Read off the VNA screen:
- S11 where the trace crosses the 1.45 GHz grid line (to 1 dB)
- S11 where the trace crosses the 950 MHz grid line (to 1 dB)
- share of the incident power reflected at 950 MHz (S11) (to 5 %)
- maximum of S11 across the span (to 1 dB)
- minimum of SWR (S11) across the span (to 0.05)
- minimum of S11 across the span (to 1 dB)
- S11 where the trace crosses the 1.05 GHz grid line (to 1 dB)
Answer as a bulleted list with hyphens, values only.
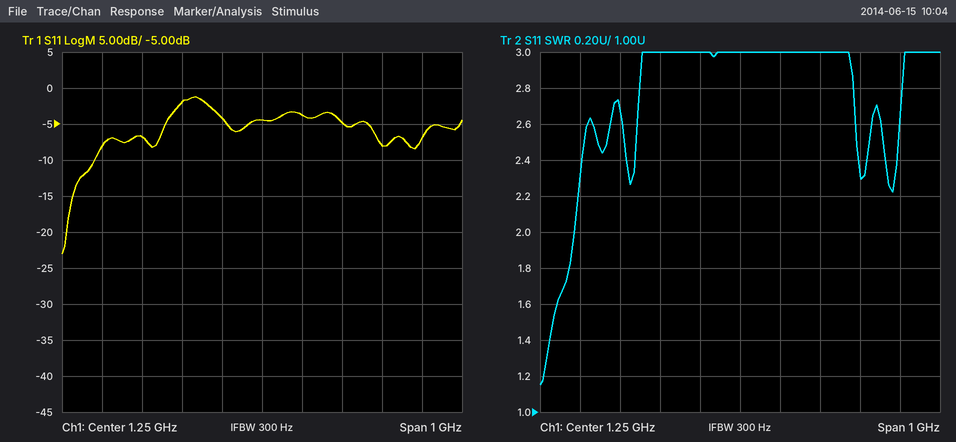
- -5 dB
- -7 dB
- 20 %
- -1 dB
- 1.15
- -23 dB
- -2 dB
